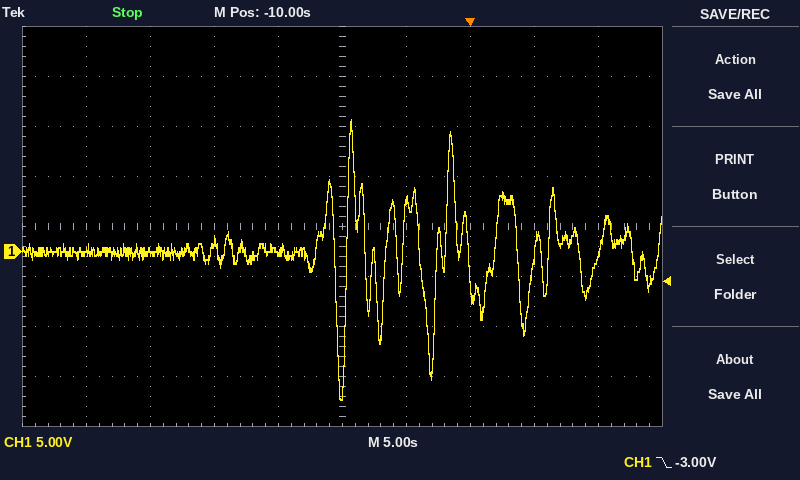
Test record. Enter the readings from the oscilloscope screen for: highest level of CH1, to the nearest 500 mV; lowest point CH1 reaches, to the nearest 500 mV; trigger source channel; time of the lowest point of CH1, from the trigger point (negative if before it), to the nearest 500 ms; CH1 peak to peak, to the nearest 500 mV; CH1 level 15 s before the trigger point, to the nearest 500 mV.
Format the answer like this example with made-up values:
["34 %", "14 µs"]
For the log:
["13.0 V", "-15.0 V", "CH1", "-10.0 s", "28.0 V", "0.0 V"]
